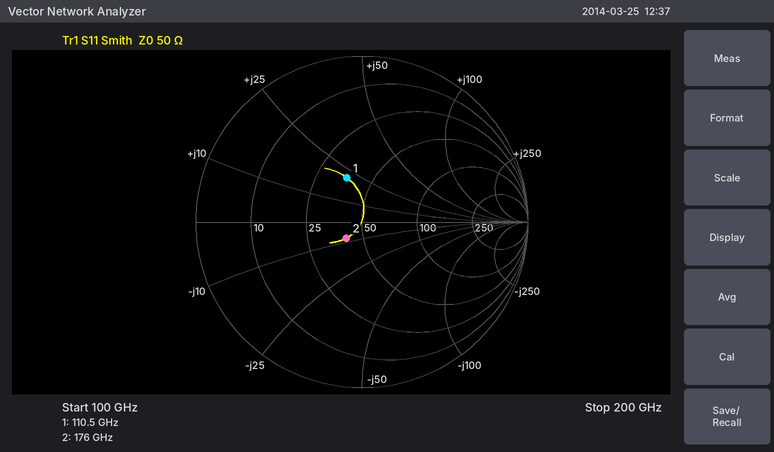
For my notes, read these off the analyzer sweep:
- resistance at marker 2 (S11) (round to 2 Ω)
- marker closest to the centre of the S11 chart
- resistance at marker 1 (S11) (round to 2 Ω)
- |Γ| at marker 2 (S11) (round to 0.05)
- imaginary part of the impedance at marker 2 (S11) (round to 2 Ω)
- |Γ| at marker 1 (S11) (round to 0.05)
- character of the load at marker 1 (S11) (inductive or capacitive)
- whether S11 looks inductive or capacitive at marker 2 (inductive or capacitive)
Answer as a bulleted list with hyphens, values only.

- 40 Ω
- marker 2
- 36 Ω
- 0.15
- -8 Ω
- 0.30
- inductive
- capacitive
